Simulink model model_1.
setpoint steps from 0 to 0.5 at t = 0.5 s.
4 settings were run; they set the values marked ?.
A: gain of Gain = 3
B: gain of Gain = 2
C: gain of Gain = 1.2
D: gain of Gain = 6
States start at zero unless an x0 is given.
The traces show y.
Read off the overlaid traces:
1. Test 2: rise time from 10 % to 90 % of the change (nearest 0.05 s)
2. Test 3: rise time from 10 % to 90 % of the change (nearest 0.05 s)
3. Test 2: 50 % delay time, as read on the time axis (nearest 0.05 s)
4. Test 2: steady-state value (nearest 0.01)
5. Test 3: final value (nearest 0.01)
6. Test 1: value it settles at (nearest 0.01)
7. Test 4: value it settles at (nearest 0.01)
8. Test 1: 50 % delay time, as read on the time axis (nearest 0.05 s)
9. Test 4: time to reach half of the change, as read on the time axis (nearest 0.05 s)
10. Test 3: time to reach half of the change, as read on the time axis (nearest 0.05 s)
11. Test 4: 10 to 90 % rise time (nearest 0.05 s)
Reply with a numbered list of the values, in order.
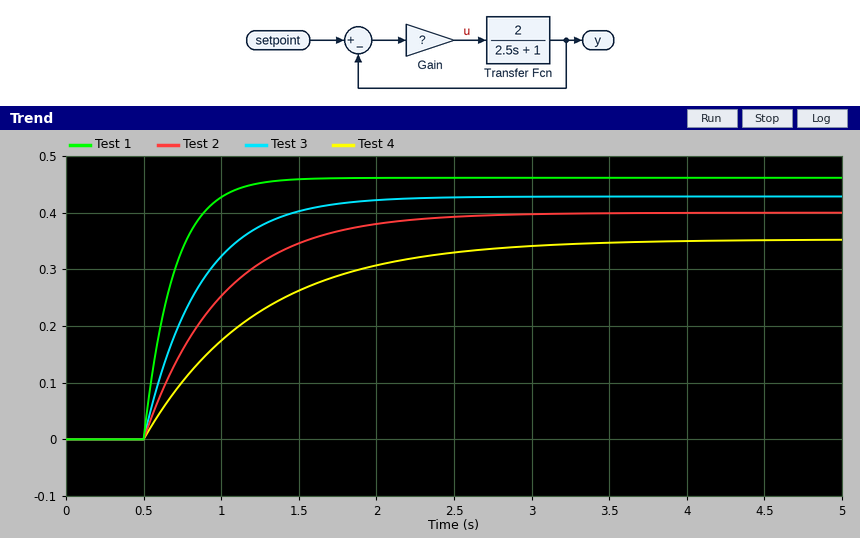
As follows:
1. 1.10 s
2. 0.80 s
3. 0.85 s
4. 0.40
5. 0.43
6. 0.46
7. 0.35
8. 0.65 s
9. 1.00 s
10. 0.75 s
11. 1.60 s
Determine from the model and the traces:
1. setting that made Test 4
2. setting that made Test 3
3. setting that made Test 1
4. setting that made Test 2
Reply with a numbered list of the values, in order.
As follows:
1. C
2. A
3. D
4. B
